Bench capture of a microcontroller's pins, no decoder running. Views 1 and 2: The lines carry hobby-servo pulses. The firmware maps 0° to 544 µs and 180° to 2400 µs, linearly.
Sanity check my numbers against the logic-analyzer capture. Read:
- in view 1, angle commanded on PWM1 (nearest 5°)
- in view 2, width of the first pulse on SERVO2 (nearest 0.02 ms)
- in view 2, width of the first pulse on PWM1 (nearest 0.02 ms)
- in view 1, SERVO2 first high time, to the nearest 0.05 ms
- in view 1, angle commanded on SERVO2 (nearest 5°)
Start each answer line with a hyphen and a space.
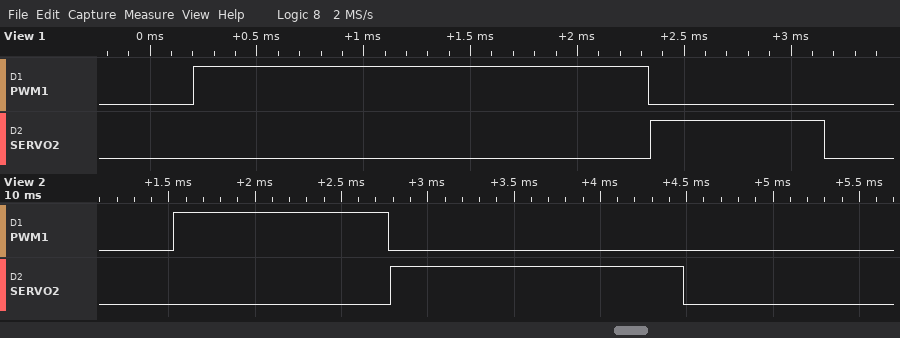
- 155°
- 1.70 ms
- 1.24 ms
- 0.80 ms
- 25°
